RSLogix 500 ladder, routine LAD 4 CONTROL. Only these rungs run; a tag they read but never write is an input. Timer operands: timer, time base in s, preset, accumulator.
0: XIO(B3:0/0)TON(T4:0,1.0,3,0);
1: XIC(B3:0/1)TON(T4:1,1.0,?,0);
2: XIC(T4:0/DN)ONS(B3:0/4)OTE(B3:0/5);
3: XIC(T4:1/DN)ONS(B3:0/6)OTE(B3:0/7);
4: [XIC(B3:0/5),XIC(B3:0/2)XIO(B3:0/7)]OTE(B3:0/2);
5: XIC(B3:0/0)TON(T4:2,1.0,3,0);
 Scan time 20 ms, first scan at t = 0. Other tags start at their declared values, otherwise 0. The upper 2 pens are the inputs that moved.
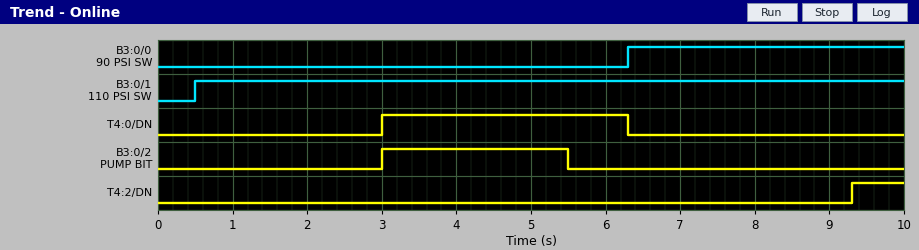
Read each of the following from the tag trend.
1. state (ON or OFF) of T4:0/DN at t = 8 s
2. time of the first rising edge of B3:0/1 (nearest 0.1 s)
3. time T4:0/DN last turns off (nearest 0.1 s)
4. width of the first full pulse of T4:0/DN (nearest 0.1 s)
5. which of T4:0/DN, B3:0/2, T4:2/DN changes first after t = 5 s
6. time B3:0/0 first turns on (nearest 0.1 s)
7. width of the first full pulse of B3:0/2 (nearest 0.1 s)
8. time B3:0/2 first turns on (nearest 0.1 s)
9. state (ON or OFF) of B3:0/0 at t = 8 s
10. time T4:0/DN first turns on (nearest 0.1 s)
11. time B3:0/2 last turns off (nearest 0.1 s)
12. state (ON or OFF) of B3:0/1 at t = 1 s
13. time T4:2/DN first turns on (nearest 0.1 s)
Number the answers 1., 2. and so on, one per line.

1. OFF
2. 0.5 s
3. 6.3 s
4. 3.3 s
5. B3:0/2
6. 6.3 s
7. 2.5 s
8. 3.0 s
9. ON
10. 3.0 s
11. 5.5 s
12. ON
13. 9.3 s
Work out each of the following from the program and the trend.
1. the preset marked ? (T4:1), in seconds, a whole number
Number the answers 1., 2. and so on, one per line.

1. 5 s
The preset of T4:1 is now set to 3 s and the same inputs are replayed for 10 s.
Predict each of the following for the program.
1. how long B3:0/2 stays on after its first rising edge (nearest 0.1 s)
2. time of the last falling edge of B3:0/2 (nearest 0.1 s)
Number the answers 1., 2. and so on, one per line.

1. 0.5 s
2. 3.5 s
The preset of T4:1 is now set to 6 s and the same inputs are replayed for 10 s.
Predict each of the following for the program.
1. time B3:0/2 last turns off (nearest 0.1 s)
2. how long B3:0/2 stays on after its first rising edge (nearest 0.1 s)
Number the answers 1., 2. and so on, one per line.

1. 6.5 s
2. 3.5 s
